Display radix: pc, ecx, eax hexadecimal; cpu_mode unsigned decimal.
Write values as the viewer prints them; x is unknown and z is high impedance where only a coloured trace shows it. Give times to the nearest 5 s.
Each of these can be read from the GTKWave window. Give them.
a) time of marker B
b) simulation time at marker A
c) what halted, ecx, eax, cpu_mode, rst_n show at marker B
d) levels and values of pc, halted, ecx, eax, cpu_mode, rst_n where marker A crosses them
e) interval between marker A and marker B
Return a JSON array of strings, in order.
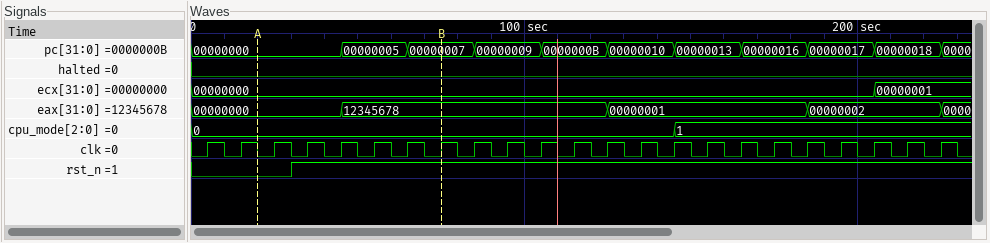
["75 s", "20 s", "halted=0, ecx=00000000, eax=12345678, cpu_mode=0, rst_n=1", "pc=00000000, halted=0, ecx=00000000, eax=00000000, cpu_mode=0, rst_n=0", "55 s"]
